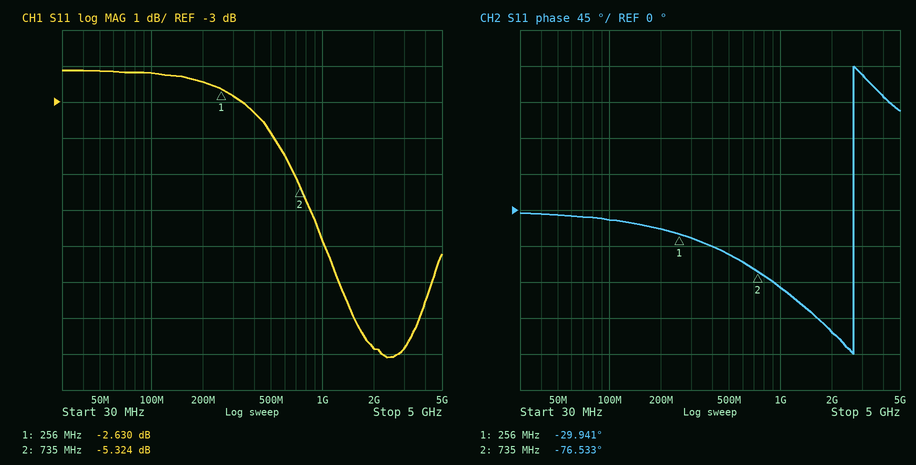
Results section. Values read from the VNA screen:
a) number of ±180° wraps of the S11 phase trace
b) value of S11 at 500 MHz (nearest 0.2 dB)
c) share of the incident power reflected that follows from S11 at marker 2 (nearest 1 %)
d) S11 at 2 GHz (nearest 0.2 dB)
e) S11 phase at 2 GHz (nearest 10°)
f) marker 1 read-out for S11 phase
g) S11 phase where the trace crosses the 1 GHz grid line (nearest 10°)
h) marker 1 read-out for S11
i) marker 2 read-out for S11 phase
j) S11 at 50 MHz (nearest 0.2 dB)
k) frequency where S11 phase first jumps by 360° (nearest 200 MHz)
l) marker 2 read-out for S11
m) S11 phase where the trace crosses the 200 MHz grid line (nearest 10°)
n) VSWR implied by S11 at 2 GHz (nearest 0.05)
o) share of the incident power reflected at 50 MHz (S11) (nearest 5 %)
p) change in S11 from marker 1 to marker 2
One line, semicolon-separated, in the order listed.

1; -3.8 dB; 29 %; -9.8 dB; -150°; -29.941°; -100°; -2.630 dB; -76.533°; -2.2 dB; 2.6 GHz; -5.324 dB; -20°; 1.95; 60 %; -2.694 dB
